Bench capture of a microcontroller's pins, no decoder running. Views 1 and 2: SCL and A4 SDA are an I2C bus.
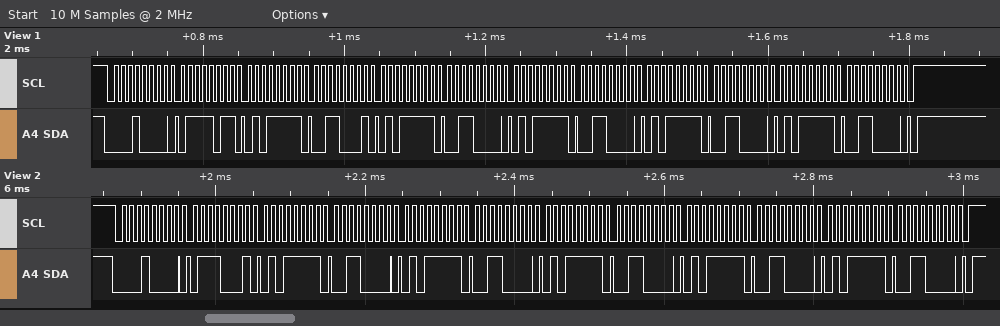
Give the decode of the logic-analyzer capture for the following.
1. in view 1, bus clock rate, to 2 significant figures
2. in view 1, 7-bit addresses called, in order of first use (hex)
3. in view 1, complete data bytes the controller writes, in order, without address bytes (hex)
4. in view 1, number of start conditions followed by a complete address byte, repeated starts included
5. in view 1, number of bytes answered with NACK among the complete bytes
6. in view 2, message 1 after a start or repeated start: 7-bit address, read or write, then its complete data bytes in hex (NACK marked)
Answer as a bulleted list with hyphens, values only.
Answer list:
- 100 kHz
- 0x08
- 7B 5F 31 5F 30 5F 30 5F 30 5F 30
- 1
- 0
- 0x08 write: 71 5F 30 5F 30 5F 30 5F 30 5F 30
